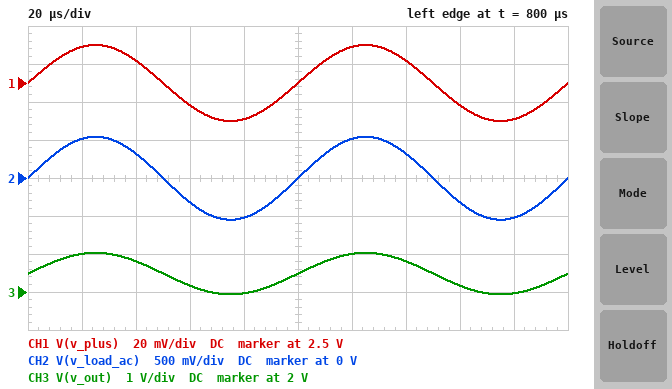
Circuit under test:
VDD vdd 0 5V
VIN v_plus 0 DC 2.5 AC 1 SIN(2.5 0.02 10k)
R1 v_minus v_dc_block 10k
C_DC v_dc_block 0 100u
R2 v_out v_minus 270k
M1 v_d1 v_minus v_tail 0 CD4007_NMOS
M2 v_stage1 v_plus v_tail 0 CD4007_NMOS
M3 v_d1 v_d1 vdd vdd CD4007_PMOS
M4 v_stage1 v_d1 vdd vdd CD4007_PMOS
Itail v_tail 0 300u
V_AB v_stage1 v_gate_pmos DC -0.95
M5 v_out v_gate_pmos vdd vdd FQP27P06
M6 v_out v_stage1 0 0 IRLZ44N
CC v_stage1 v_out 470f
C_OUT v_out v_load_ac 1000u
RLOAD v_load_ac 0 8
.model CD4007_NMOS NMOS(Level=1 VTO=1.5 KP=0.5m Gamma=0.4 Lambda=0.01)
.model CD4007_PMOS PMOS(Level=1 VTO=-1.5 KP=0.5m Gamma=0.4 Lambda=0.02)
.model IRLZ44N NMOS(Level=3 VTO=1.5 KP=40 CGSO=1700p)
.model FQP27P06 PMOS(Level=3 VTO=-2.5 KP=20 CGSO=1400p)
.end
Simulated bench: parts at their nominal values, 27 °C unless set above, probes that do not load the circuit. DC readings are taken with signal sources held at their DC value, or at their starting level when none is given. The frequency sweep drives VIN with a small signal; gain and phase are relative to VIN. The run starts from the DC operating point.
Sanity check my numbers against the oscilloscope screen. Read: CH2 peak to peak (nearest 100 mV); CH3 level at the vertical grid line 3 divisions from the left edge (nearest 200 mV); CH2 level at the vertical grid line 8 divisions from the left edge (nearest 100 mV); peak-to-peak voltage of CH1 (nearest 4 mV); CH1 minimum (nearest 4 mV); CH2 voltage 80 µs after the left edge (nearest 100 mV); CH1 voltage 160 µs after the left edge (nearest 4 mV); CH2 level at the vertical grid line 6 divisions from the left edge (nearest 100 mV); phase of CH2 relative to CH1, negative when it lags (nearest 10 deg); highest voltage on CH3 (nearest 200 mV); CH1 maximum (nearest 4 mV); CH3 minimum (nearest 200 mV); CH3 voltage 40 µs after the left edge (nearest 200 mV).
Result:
1.1 V
2.2 V
-300 mV
40 mV
2.480 V
-500 mV
2.488 V
500 mV
0 deg
3.0 V
2.520 V
2.0 V
2.8 V
